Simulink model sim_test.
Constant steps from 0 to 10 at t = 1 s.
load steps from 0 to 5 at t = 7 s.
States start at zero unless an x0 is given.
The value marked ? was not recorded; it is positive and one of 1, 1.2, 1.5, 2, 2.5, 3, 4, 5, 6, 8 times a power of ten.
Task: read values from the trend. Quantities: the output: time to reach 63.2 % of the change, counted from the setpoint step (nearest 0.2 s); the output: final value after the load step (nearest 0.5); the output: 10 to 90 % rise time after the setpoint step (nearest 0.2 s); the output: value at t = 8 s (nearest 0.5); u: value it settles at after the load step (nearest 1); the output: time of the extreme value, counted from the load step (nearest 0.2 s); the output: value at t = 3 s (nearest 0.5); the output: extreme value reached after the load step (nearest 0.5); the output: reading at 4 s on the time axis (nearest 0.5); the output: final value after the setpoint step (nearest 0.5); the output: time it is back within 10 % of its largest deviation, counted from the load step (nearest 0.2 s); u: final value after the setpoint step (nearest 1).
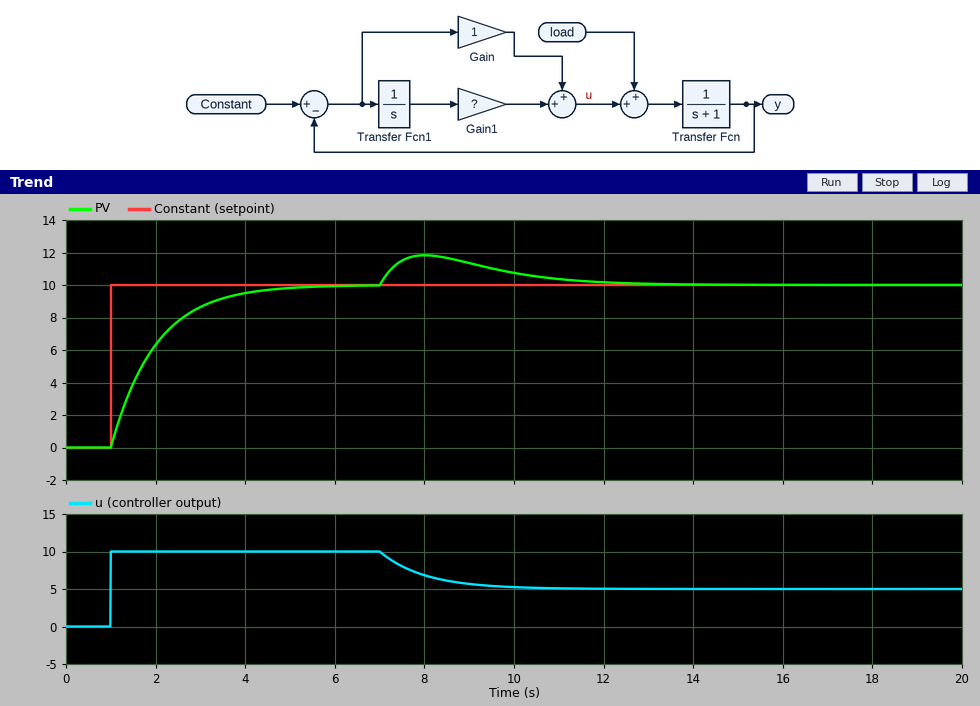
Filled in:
1.0 s
10.0
2.2 s
12.0
5
1.0 s
8.5
12.0
9.5
10.0
4.8 s
10
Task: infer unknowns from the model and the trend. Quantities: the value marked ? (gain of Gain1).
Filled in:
1
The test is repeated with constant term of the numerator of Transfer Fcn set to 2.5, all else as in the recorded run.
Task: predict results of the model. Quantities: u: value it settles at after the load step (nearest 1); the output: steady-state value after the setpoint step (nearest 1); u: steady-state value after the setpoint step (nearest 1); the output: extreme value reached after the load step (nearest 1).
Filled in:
-1
10
4
13
